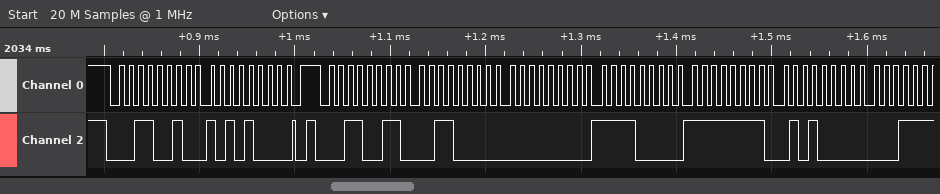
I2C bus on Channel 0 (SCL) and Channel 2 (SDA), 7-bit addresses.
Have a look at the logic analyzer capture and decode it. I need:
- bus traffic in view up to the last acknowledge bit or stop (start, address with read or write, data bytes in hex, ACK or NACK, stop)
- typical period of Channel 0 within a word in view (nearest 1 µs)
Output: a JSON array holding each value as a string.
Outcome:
["start, address 19 write ACK, A8 ACK, stop, start, address 19 read ACK, 30 ACK, 00 ACK, F0 ACK, FF ACK, 50 ACK", "10 µs"]
